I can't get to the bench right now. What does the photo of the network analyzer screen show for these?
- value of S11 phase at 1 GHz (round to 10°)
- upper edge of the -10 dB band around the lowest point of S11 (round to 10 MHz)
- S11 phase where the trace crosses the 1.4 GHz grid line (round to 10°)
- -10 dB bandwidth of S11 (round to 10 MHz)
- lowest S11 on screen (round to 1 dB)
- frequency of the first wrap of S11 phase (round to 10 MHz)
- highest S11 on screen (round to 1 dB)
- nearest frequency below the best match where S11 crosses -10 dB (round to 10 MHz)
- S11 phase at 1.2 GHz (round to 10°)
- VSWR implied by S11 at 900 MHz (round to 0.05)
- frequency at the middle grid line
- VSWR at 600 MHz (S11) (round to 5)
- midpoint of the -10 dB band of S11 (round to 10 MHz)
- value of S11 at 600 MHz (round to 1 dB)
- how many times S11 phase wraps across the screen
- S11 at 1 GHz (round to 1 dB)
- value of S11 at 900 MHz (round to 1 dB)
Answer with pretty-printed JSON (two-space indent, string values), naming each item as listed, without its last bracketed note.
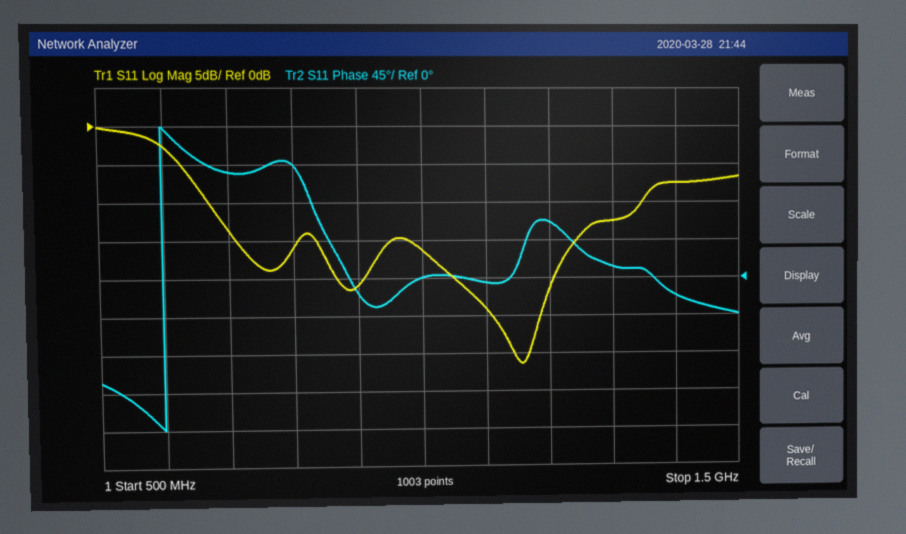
{
  "value of S11 phase at 1 GHz": "0°",
  "upper edge of the -10 dB band around the lowest point of S11": "1.35 GHz",
  "S11 phase where the trace crosses the 1.4 GHz grid line": "-20°",
  "-10 dB bandwidth of S11": "680 MHz",
  "lowest S11 on screen": "-31 dB",
  "frequency of the first wrap of S11 phase": "600 MHz",
  "highest S11 on screen": "0 dB",
  "nearest frequency below the best match where S11 crosses -10 dB": "670 MHz",
  "S11 phase at 1.2 GHz": "70°",
  "VSWR implied by S11 at 900 MHz": "1.20",
  "frequency at the middle grid line": "1 GHz",
  "VSWR at 600 MHz (S11)": "5",
  "midpoint of the -10 dB band of S11": "1.01 GHz",
  "value of S11 at 600 MHz": "-3 dB",
  "how many times S11 phase wraps across the screen": "1",
  "S11 at 1 GHz": "-16 dB",
  "value of S11 at 900 MHz": "-21 dB"
}
